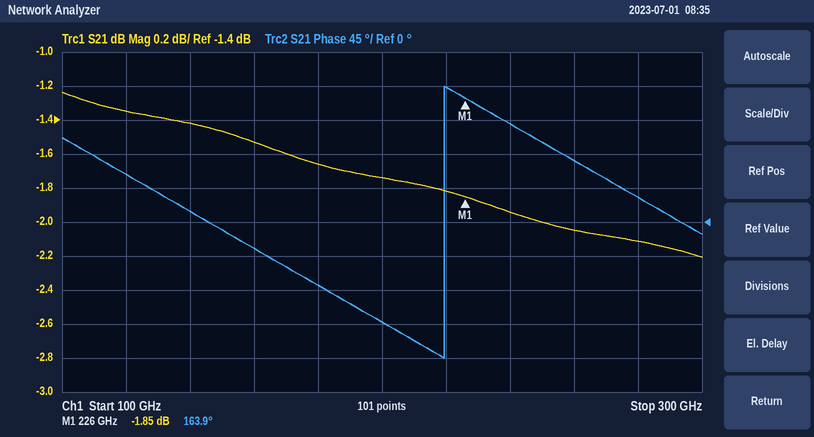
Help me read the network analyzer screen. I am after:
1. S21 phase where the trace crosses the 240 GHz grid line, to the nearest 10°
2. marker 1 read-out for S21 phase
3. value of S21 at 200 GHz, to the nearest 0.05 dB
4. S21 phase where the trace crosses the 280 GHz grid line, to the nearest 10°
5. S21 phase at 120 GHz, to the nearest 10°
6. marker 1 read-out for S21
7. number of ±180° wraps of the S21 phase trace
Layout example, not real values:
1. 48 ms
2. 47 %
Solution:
1. 130°
2. 163.9°
3. -1.75 dB
4. 30°
5. 60°
6. -1.85 dB
7. 1
